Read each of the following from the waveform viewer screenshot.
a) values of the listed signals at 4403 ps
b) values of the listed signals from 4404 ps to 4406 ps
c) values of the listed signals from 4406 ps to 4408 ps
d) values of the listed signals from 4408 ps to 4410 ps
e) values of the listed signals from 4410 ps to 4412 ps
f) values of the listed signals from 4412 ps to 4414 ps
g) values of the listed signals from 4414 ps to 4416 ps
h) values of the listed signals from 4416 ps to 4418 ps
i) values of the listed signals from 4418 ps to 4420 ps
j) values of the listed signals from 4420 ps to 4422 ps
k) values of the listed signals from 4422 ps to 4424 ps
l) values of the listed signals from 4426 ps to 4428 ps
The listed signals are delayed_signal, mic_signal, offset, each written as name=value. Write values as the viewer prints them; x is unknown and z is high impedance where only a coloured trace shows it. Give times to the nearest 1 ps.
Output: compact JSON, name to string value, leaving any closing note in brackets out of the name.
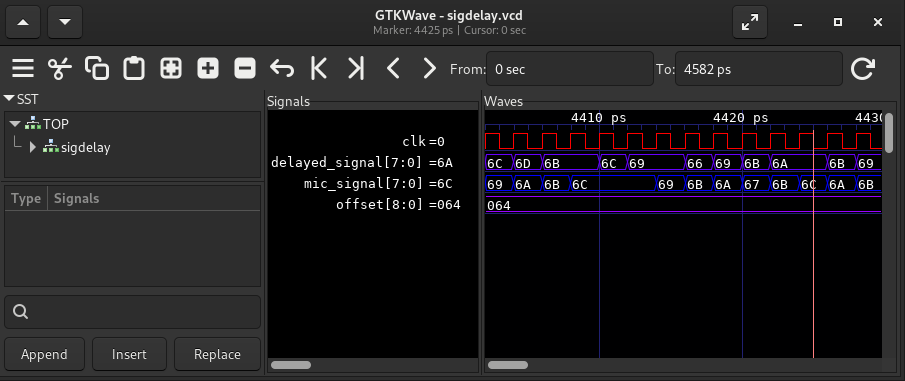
{"values of the listed signals at 4403 ps": "delayed_signal=6C, mic_signal=69, offset=064", "values of the listed signals from 4404 ps to 4406 ps": "delayed_signal=6D, mic_signal=6A, offset=064", "values of the listed signals from 4406 ps to 4408 ps": "delayed_signal=6B, mic_signal=6B, offset=064", "values of the listed signals from 4408 ps to 4410 ps": "delayed_signal=6B, mic_signal=6C, offset=064", "values of the listed signals from 4410 ps to 4412 ps": "delayed_signal=6C, mic_signal=6C, offset=064", "values of the listed signals from 4412 ps to 4414 ps": "delayed_signal=69, mic_signal=6C, offset=064", "values of the listed signals from 4414 ps to 4416 ps": "delayed_signal=69, mic_signal=69, offset=064", "values of the listed signals from 4416 ps to 4418 ps": "delayed_signal=66, mic_signal=6B, offset=064", "values of the listed signals from 4418 ps to 4420 ps": "delayed_signal=69, mic_signal=6A, offset=064", "values of the listed signals from 4420 ps to 4422 ps": "delayed_signal=6B, mic_signal=67, offset=064", "values of the listed signals from 4422 ps to 4424 ps": "delayed_signal=6A, mic_signal=6B, offset=064", "values of the listed signals from 4426 ps to 4428 ps": "delayed_signal=6B, mic_signal=6A, offset=064"}
